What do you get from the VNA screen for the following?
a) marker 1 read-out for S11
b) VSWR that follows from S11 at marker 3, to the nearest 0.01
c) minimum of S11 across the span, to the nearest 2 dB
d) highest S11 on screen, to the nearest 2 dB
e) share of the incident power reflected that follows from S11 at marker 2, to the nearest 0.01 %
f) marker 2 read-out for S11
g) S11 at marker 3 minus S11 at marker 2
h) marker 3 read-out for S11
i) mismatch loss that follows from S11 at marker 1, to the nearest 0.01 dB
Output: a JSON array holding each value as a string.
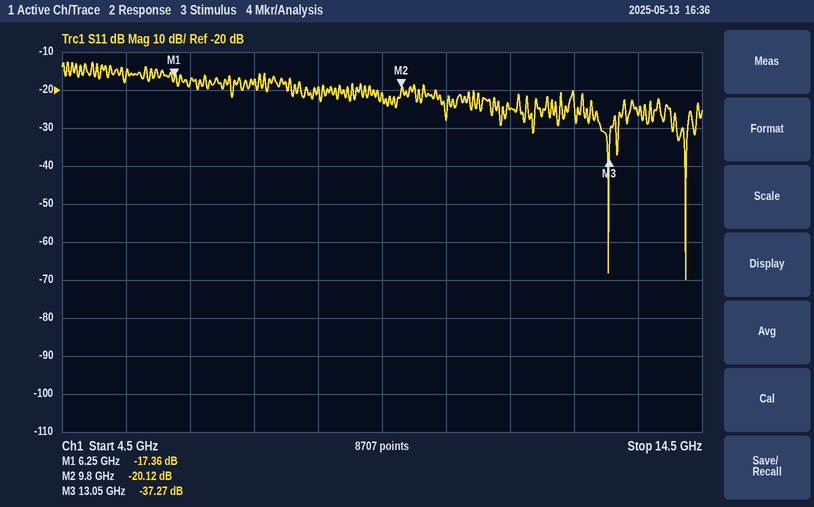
["-17.36 dB", "1.03", "-70 dB", "-12 dB", "0.97 %", "-20.12 dB", "-17.15 dB", "-37.27 dB", "0.08 dB"]
